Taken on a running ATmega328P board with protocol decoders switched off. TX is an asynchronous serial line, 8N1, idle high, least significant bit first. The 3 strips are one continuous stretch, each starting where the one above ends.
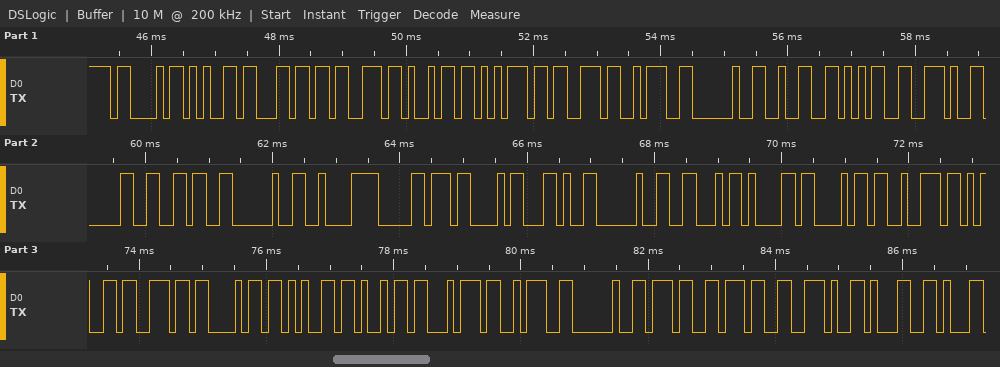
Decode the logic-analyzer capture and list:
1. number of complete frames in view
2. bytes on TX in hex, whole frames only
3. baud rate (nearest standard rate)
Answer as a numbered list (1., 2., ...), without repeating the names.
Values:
1. 36
2. 0x43 0x65 0x6C 0x73 0x69 0x75 0x73 0x3A 0x20 0x32 0x35 0x2E 0x30 0x36 0x20 0xC2 0xB0 0x43 0x2C 0x20 0x46 0x61 0x68 0x72 0x65 0x6E 0x68 0x65 0x69 0x74 0x3A 0x20 0x37 0x37 0x2E 0x31
3. 9600 baud
